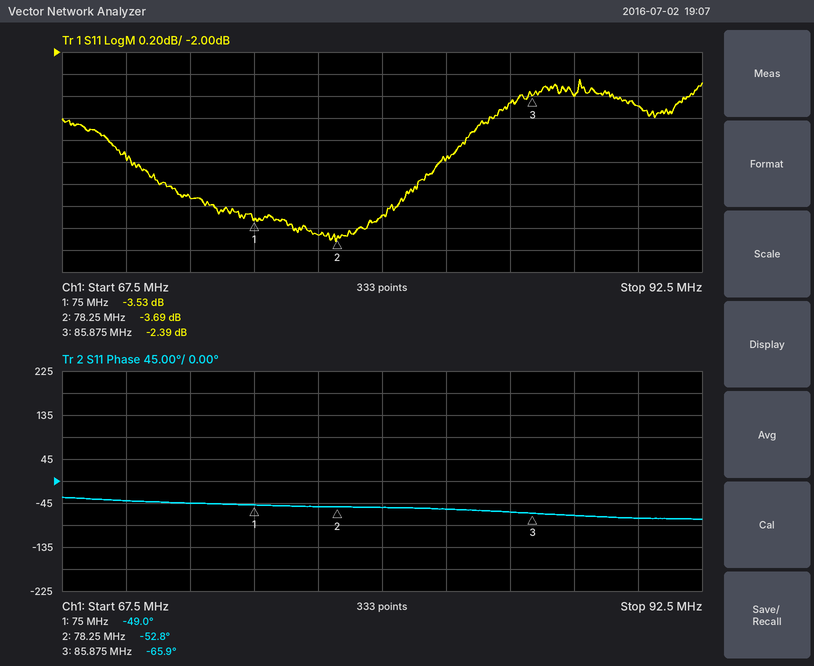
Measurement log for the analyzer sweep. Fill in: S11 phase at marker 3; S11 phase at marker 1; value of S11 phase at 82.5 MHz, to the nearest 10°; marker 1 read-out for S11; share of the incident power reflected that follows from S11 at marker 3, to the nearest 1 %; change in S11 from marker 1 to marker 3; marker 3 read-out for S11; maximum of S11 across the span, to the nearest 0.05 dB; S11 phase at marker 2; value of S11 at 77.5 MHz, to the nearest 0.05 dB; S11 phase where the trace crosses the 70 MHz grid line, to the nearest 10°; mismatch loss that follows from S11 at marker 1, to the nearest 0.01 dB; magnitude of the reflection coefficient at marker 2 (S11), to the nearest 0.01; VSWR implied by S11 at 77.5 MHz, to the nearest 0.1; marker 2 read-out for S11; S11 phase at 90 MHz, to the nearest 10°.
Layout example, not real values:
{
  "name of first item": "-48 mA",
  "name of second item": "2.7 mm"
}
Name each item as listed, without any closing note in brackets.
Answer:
{
  "S11 phase at marker 3": "-65.9°",
  "S11 phase at marker 1": "-49.0°",
  "value of S11 phase at 82.5 MHz, to the nearest 10°": "-60°",
  "marker 1 read-out for S11": "-3.53 dB",
  "share of the incident power reflected that follows from S11 at marker 3, to the nearest 1 %": "58 %",
  "change in S11 from marker 1 to marker 3": "1.14 dB",
  "marker 3 read-out for S11": "-2.39 dB",
  "maximum of S11 across the span, to the nearest 0.05 dB": "-2.25 dB",
  "S11 phase at marker 2": "-52.8°",
  "value of S11 at 77.5 MHz, to the nearest 0.05 dB": "-3.65 dB",
  "S11 phase where the trace crosses the 70 MHz grid line, to the nearest 10°": "-40°",
  "mismatch loss that follows from S11 at marker 1, to the nearest 0.01 dB": "2.55 dB",
  "magnitude of the reflection coefficient at marker 2 (S11), to the nearest 0.01": "0.65",
  "VSWR implied by S11 at 77.5 MHz, to the nearest 0.1": "4.8",
  "marker 2 read-out for S11": "-3.69 dB",
  "S11 phase at 90 MHz, to the nearest 10°": "-80°"
}
